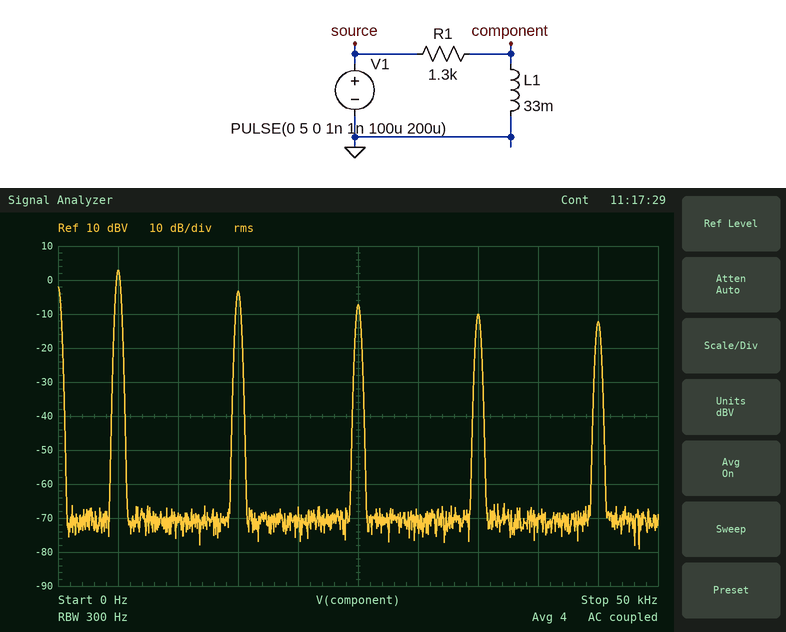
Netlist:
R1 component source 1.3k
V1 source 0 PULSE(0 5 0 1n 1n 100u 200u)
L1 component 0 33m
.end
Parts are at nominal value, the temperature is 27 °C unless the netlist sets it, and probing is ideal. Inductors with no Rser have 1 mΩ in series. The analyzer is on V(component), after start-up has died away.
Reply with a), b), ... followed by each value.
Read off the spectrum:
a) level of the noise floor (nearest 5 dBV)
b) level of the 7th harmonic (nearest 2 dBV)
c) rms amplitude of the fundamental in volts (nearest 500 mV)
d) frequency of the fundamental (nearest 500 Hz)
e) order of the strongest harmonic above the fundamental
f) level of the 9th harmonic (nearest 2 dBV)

a) -70 dBV
b) -10 dBV
c) 1.5 V
d) 5.0 kHz
e) 3
f) -12 dBV
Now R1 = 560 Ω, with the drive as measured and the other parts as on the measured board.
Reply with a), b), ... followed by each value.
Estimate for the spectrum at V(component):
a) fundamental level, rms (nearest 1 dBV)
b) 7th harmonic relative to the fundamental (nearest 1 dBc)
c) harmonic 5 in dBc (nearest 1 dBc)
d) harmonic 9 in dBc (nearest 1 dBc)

a) 6 dBV
b) -16 dBc
c) -13 dBc
d) -18 dBc
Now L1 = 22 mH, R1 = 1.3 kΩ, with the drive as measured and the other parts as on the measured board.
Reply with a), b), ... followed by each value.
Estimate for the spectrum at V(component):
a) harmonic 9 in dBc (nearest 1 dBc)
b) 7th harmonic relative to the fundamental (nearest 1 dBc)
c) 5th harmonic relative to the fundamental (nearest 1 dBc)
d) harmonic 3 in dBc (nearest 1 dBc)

a) -13 dBc
b) -11 dBc
c) -8 dBc
d) -4 dBc
